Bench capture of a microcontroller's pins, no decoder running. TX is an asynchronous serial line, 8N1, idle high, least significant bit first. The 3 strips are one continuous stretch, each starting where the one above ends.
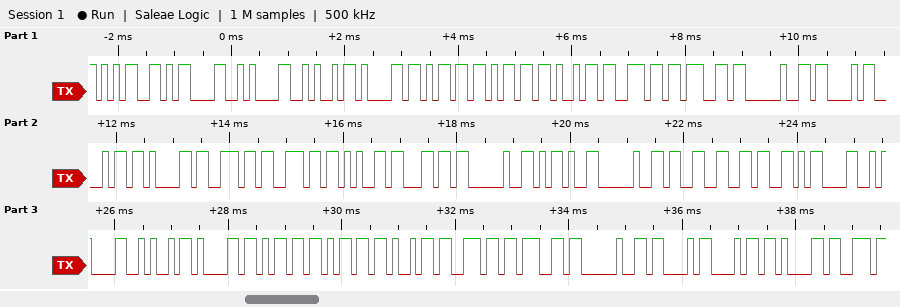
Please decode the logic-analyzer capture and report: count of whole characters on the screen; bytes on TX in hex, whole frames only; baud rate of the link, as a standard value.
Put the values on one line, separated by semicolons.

36; 35 0D 0A 4A 61 6D 6D 69 6E 67 20 43 68 61 6E 6E 65 6C 20 2D 20 33 36 0D 0A 4A 61 6D 6D 69 6E 67 20 43 68 61; 9600 baud
